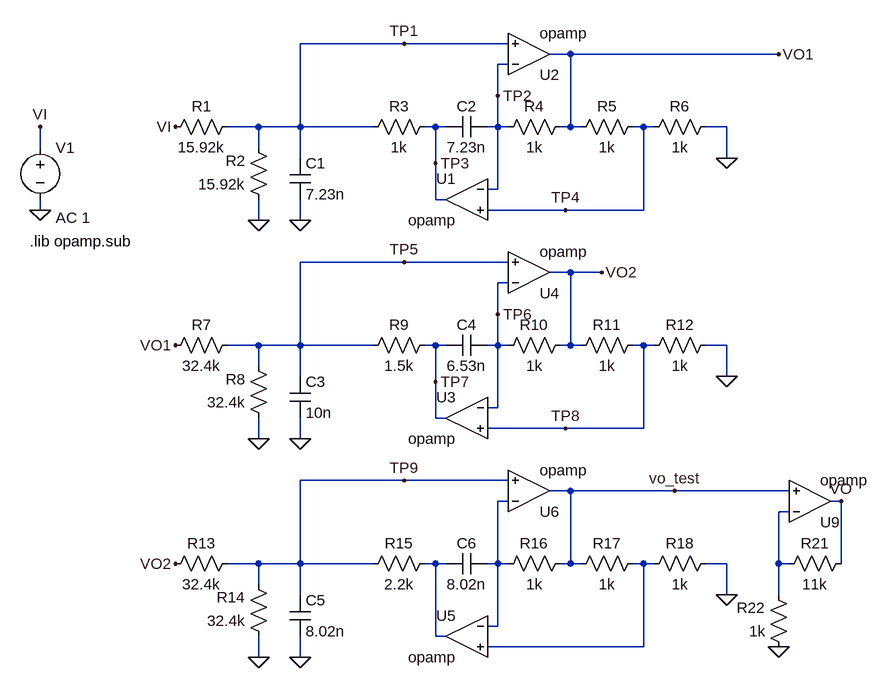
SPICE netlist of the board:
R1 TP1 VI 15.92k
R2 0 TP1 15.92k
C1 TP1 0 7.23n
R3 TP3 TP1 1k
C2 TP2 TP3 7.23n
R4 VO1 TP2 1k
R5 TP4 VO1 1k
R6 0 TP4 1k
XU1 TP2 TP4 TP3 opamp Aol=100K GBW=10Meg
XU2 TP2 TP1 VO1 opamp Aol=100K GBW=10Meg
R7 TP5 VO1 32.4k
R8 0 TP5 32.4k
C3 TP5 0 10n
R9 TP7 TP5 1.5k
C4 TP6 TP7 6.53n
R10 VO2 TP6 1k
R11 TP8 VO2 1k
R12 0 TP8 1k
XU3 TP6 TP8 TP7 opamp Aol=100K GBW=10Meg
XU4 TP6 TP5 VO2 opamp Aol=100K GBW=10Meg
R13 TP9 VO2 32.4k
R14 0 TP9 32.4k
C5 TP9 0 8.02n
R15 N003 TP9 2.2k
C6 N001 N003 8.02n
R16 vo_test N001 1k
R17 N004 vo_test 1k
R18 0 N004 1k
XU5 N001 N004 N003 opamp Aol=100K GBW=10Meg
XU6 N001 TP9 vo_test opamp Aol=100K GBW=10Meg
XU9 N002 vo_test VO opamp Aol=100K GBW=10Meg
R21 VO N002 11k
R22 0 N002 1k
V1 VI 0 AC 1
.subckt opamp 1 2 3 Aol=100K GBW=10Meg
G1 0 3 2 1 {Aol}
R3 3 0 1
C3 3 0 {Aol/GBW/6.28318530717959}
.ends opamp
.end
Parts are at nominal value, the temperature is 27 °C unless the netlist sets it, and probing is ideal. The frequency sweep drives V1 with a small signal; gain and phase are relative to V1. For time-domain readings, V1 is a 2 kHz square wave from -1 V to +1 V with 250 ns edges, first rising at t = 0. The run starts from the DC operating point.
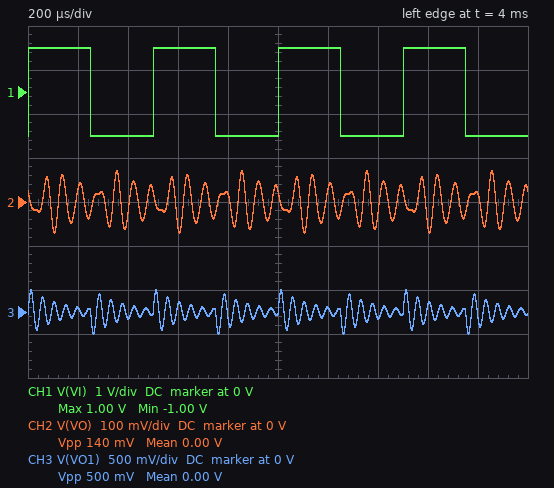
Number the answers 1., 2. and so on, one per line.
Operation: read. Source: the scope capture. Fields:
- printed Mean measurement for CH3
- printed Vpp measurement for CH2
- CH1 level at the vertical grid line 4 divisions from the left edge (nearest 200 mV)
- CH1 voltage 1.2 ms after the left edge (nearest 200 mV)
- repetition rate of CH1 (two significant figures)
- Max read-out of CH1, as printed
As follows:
1. 0.00 V
2. 140 mV
3. -1.0 V
4. 1.0 V
5. 2.0 kHz
6. 1.00 V
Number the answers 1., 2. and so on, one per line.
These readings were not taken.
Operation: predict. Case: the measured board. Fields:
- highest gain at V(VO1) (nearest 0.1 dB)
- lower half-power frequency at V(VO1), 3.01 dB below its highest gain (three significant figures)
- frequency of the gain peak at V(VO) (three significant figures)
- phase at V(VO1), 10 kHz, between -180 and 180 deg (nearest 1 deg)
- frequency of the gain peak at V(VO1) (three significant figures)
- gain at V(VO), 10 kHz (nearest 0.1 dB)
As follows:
1. 0 dB
2. 20.6 kHz
3. 16.0 kHz
4. 86 deg
5. 21.9 kHz
6. -41.6 dB
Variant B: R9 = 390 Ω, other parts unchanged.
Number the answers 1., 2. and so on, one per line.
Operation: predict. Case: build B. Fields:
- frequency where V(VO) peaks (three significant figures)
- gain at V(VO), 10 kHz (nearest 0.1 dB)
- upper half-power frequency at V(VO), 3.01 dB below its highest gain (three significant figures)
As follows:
1. 31.3 kHz
2. -56.6 dB
3. 31.8 kHz
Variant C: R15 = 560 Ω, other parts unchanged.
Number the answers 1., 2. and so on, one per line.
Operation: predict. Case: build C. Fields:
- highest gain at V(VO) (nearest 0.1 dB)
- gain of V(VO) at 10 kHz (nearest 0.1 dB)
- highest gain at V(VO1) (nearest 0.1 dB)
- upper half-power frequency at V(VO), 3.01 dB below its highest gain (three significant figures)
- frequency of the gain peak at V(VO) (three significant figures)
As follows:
1. -12.9 dB
2. -59.2 dB
3. 0 dB
4. 26.8 kHz
5. 26.3 kHz
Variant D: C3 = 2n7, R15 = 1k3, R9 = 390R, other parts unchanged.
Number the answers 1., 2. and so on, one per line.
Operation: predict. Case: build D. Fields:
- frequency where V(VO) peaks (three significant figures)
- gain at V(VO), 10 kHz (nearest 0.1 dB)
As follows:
1. 17.5 kHz
2. -65.5 dB
